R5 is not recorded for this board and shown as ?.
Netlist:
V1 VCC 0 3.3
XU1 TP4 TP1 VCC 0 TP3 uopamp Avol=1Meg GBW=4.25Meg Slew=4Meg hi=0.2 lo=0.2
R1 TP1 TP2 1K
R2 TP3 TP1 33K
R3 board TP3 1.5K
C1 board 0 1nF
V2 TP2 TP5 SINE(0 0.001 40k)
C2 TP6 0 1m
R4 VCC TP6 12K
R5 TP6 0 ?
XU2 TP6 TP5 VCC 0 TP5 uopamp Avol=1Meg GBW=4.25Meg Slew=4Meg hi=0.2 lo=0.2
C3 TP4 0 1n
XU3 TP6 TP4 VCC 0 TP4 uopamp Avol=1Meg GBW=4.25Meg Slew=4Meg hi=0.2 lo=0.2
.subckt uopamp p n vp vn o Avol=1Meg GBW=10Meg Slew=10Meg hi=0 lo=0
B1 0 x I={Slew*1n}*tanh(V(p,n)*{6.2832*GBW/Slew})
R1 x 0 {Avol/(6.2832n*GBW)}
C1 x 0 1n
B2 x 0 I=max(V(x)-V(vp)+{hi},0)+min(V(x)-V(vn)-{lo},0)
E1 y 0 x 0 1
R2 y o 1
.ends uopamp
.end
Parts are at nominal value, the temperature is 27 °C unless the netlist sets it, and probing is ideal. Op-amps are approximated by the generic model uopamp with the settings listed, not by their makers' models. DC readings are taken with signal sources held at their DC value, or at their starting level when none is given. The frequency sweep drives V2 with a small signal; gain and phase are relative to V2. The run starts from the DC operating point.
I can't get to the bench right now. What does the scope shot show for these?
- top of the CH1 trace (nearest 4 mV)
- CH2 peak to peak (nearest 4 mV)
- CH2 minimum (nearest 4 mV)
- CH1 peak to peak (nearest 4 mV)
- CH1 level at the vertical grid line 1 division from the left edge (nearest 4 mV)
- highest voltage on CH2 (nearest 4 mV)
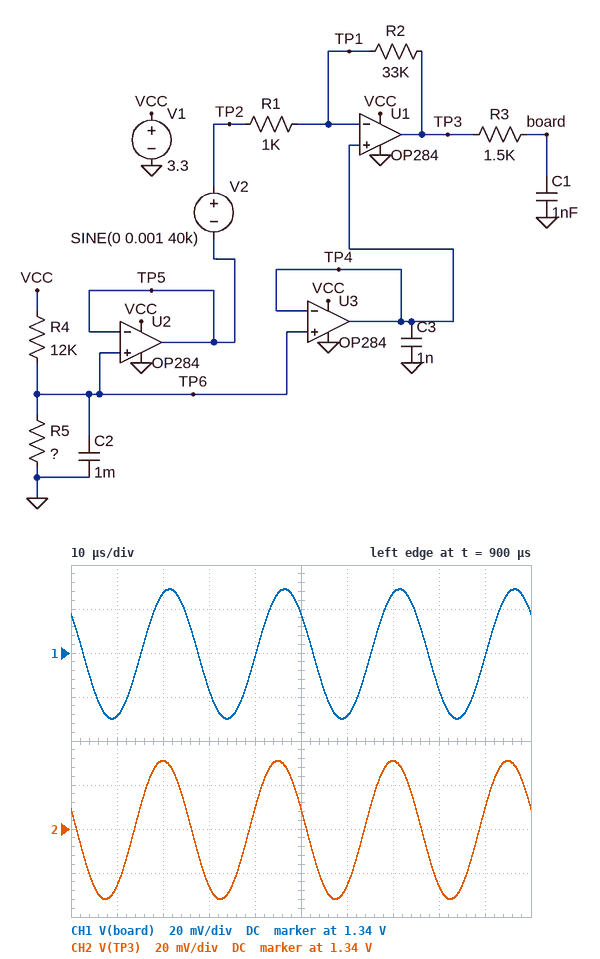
1.368 V
64 mV
1.308 V
60 mV
1.312 V
1.372 V
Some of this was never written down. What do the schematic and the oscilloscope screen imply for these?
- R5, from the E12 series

8.2 kΩ
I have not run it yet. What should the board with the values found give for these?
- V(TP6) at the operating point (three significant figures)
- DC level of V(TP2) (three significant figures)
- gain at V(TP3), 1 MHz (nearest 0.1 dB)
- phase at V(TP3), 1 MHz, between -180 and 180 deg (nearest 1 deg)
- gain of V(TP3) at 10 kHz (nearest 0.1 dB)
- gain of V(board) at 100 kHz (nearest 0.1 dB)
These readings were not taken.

1.34 V
1.34 V
12.2 dB
97 deg
30.3 dB
25.5 dB
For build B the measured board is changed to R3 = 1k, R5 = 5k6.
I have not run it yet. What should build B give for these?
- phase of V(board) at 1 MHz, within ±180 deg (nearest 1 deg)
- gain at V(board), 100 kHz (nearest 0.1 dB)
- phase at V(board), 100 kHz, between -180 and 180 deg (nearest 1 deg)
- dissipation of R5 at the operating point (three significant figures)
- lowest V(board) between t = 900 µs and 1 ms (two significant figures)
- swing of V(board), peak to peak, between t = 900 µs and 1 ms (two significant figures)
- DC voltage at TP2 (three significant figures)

16 deg
26.8 dB
109 deg
197 µW
1.0 V
61 mV
1.05 V
